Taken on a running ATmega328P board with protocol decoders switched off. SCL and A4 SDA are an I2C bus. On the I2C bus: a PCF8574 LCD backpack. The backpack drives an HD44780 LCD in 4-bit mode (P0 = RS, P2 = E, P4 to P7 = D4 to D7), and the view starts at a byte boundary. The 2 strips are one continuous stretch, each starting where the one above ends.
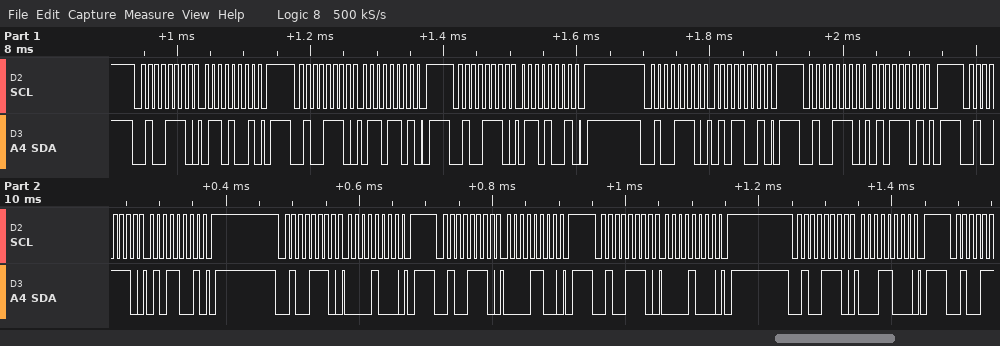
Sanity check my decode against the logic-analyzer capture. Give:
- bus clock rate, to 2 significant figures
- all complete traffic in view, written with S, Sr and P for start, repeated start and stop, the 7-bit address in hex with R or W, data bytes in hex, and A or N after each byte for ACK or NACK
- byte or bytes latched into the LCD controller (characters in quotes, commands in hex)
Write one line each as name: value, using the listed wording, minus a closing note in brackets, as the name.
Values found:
bus clock rate, to 2 significant figures: 100 kHz
all complete traffic in view, written with S, Sr and P for start, repeated start and stop, the 7-bit address in hex with R or W, data bytes in hex, and A or N after each byte for ACK or NACK: S 27W A 69 A P S 27W A 6D A P S 27W A 69 A P S 27W A 59 A P S 27W A 5D A P S 27W A 59 A P S 27W A 08 A P S 27W A 0C A P S 27W A 08 A P S 27W A 18 A P
byte or bytes latched into the LCD controller: 'e'
